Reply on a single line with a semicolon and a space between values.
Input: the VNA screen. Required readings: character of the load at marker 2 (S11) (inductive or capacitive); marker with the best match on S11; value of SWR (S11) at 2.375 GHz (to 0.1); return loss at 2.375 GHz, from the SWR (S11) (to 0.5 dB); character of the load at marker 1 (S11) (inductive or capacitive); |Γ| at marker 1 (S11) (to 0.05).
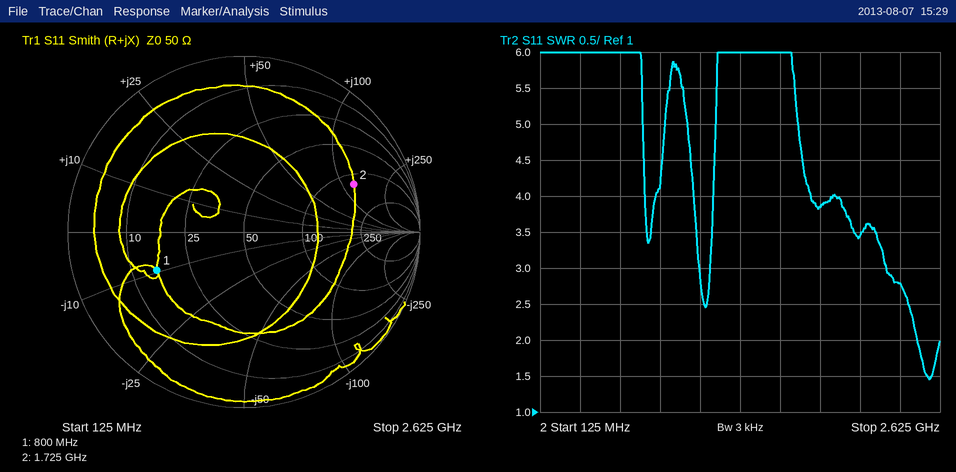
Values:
inductive; marker 1; 2.8; 6.5 dB; capacitive; 0.55
